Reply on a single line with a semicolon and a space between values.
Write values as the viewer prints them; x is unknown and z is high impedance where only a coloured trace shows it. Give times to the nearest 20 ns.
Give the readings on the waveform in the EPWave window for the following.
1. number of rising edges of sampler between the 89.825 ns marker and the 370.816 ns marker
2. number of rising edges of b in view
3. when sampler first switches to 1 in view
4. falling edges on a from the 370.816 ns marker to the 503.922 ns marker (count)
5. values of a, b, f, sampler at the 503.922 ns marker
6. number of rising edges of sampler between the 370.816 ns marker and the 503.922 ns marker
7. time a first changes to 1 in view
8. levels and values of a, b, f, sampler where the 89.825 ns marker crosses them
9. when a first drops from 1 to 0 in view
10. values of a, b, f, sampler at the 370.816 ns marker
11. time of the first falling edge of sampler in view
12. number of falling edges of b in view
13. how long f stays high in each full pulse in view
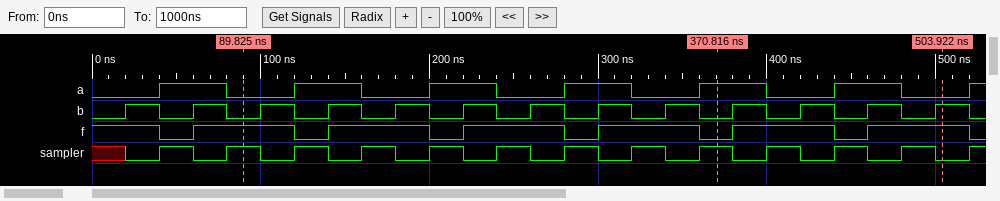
7; 13; 40 ns; 2; a=0, b=1, f=1, sampler=0; 3; 40 ns; a=0, b=0, f=1, sampler=1; 80 ns; a=1, b=0, f=0, sampler=1; 60 ns; 13; 60 ns, 60 ns, 60 ns, 60 ns, 60 ns, 60 ns
